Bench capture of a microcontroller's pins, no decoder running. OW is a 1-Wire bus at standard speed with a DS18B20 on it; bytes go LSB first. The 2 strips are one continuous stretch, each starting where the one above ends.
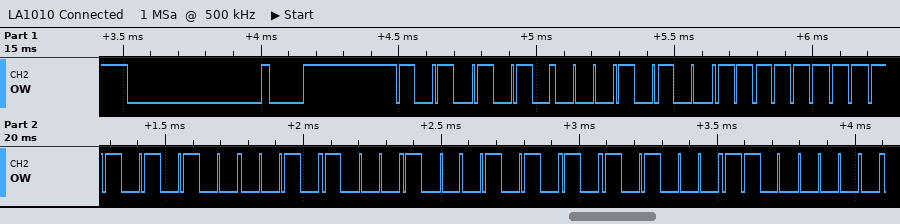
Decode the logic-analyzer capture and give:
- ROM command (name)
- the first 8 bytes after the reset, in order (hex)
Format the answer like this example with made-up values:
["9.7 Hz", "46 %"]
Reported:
["Match ROM", "55 28 FF 2B 14 51 15 03"]
